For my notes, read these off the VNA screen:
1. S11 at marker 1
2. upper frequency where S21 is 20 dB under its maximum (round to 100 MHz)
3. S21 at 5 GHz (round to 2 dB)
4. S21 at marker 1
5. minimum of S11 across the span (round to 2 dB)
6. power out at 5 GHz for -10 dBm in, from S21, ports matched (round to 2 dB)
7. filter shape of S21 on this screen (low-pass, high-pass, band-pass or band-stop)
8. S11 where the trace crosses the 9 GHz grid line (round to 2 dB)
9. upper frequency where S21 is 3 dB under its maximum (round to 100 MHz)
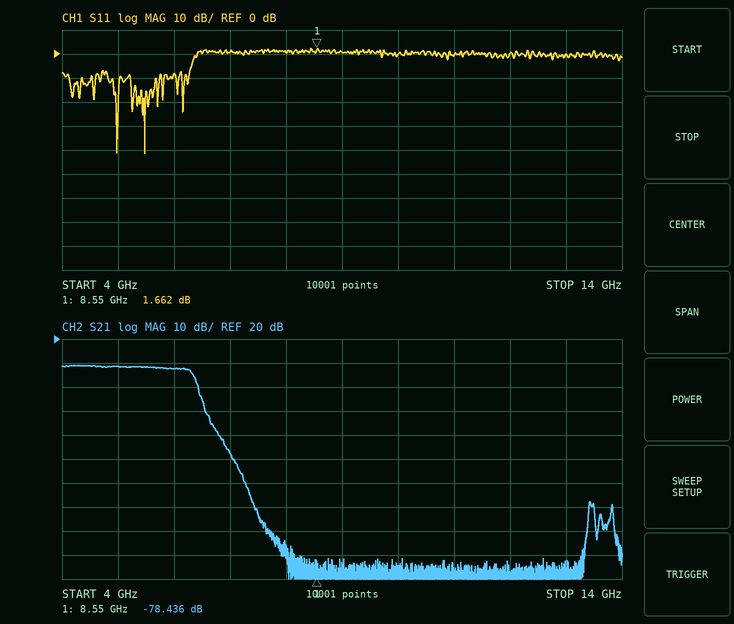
1.662 dB
6.6 GHz
8 dB
-78.436 dB
-42 dB
-2 dBm
low-pass
0 dB
6.3 GHz
